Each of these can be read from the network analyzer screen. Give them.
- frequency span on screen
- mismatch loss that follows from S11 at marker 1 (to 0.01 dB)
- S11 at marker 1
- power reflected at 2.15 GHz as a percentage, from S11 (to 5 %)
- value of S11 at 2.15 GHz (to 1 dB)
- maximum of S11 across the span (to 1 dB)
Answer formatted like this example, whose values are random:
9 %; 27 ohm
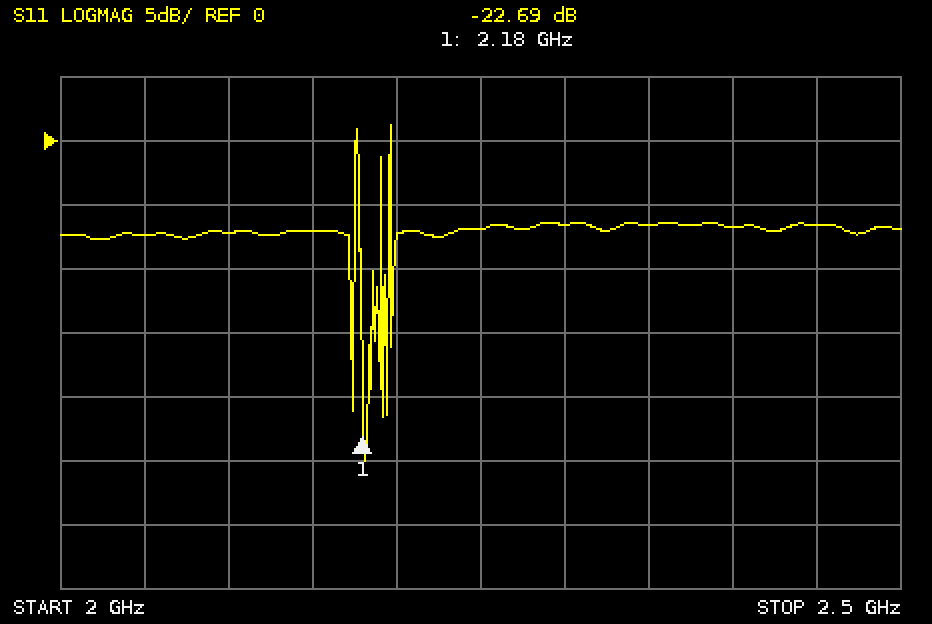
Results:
500 MHz; 0.02 dB; -22.69 dB; 20 %; -7 dB; 1 dB
